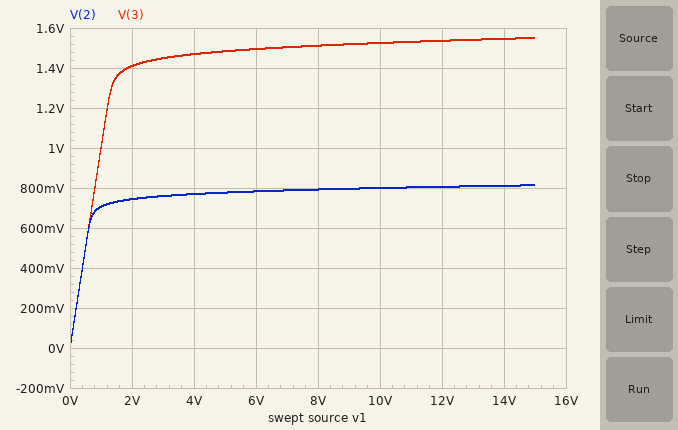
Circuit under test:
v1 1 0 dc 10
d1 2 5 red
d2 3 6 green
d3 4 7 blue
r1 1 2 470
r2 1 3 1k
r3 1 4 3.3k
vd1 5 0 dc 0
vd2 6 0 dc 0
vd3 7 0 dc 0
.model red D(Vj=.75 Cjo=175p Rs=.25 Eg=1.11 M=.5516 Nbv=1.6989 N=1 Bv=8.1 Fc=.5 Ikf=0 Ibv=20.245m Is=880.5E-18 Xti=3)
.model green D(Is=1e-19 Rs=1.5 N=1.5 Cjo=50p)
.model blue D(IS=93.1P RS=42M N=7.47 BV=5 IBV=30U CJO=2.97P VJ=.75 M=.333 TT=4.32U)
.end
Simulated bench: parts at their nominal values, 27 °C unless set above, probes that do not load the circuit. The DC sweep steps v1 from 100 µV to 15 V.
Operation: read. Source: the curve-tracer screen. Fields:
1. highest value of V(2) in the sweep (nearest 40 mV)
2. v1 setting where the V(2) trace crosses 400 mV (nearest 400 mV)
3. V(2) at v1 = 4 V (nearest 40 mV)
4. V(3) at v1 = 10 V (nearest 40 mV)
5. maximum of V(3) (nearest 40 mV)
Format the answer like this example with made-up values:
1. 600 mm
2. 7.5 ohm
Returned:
1. 800 mV
2. 400 mV
3. 760 mV
4. 1.52 V
5. 1.56 V
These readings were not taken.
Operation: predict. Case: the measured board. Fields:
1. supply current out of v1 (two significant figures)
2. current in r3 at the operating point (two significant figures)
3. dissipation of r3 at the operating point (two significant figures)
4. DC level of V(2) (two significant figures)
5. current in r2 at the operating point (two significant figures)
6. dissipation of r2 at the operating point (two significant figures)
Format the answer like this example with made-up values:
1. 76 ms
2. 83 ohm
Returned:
1. 30 mA
2. 2.0 mA
3. 14 mW
4. 800 mV
5. 8.5 mA
6. 72 mW
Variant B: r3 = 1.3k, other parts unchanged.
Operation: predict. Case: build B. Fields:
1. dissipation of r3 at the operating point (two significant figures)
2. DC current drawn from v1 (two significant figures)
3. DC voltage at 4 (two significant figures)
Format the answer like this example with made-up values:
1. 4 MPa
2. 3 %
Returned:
1. 33 mW
2. 33 mA
3. 3.4 V
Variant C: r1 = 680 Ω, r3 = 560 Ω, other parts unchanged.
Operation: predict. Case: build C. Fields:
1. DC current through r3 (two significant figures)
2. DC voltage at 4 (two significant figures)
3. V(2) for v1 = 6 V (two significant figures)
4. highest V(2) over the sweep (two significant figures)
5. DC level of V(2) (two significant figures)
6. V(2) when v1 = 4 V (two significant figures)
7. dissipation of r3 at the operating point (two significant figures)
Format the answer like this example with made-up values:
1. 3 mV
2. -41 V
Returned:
1. 11 mA
2. 3.6 V
3. 770 mV
4. 800 mV
5. 790 mV
6. 760 mV
7. 73 mW
